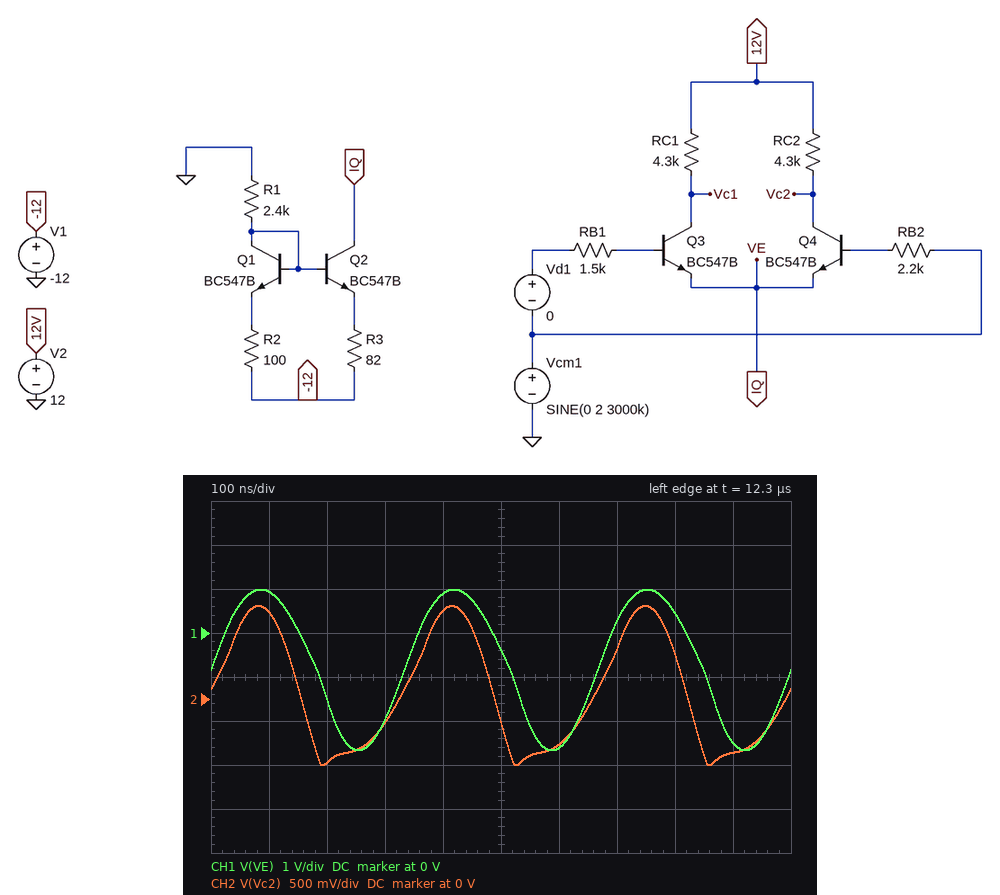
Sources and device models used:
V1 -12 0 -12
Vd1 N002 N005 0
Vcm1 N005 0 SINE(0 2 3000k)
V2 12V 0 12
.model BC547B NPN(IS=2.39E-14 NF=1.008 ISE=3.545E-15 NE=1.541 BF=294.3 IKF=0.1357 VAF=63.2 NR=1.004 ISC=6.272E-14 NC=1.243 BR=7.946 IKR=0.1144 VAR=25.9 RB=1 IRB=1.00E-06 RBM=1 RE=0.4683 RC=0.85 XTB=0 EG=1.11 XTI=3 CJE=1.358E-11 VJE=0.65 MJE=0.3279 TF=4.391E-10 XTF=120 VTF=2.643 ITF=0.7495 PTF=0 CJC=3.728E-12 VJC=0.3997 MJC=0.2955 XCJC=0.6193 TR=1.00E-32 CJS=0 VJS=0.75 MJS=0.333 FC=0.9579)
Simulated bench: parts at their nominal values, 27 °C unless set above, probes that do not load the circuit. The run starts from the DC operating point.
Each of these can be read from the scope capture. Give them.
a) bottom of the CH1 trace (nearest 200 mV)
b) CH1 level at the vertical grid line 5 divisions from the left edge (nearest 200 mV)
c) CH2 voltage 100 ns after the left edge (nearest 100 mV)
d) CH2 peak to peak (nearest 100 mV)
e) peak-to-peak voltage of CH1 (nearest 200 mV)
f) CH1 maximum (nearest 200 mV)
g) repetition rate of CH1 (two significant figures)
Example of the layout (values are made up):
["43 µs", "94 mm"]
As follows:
["-2.6 V", "-400 mV", "1.0 V", "1.8 V", "3.6 V", "1.0 V", "3.0 MHz"]
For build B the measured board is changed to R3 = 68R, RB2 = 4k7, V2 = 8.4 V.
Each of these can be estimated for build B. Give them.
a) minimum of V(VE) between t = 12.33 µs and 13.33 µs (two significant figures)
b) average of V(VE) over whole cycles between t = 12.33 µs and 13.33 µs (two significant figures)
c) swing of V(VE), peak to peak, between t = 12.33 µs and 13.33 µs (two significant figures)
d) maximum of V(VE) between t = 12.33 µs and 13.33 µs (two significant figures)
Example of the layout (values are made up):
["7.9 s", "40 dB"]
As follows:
["-3.7 V", "-2.4 V", "2.6 V", "-1.1 V"]
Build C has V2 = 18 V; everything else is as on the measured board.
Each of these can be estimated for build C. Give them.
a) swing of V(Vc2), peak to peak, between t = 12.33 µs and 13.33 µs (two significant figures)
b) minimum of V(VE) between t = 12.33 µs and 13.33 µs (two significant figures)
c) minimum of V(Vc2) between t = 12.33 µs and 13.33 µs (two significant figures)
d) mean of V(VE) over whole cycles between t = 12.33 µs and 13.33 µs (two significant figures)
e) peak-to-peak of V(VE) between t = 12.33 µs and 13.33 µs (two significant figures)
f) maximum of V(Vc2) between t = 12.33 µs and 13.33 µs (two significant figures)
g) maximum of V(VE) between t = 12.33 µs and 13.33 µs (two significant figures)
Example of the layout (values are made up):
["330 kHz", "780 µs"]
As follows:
["510 mV", "-2.7 V", "6.7 V", "-680 mV", "4.0 V", "7.2 V", "1.3 V"]
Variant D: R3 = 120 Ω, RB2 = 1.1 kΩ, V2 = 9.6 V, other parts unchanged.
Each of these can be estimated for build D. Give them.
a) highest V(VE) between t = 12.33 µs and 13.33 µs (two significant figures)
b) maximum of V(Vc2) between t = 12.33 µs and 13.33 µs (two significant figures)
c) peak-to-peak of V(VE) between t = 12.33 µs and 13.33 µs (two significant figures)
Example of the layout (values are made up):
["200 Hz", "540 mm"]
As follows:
["1.3 V", "1.4 V", "3.9 V"]
